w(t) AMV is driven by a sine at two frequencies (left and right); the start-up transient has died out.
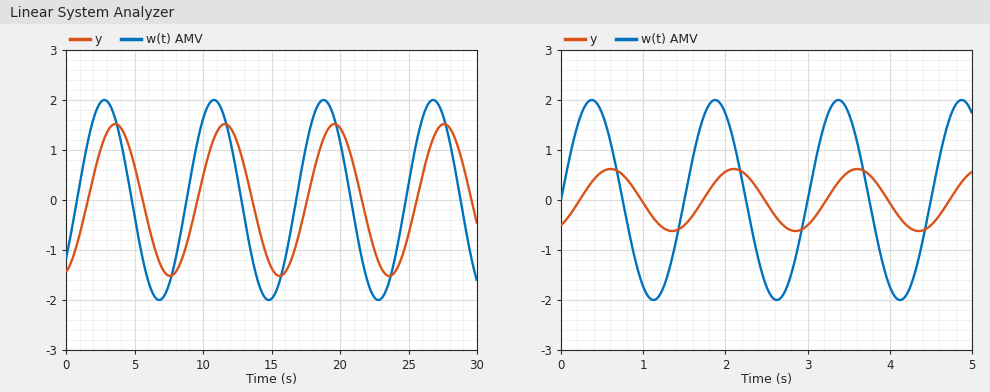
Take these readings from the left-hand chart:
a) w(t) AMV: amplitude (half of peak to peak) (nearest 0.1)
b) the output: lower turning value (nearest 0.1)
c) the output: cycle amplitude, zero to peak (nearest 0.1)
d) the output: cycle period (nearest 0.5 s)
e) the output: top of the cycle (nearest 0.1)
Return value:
2.0
-1.5
1.5
8.0 s
1.5
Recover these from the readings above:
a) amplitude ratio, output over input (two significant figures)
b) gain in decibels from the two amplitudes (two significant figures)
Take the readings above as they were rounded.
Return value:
0.75
-2.5 dB
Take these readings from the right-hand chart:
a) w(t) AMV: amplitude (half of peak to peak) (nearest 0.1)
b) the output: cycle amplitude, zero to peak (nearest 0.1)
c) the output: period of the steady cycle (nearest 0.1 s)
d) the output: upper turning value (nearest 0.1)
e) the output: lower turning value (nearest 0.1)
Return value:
2.0
0.6
1.5 s
0.6
-0.6
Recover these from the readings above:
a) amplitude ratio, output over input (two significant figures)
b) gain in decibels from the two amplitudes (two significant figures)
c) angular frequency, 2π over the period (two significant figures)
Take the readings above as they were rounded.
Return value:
0.30
-10 dB
4.2 rad/s
